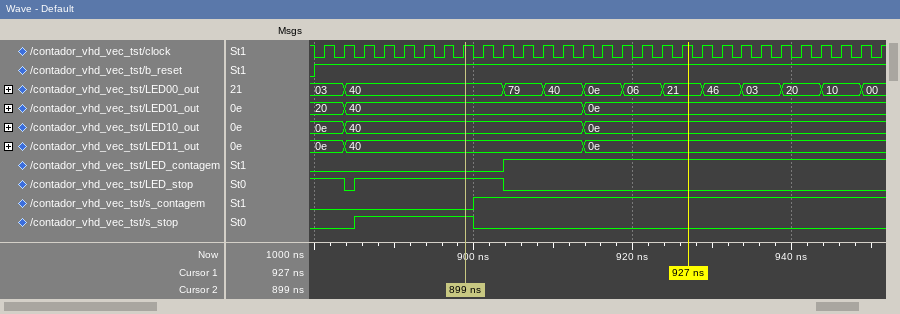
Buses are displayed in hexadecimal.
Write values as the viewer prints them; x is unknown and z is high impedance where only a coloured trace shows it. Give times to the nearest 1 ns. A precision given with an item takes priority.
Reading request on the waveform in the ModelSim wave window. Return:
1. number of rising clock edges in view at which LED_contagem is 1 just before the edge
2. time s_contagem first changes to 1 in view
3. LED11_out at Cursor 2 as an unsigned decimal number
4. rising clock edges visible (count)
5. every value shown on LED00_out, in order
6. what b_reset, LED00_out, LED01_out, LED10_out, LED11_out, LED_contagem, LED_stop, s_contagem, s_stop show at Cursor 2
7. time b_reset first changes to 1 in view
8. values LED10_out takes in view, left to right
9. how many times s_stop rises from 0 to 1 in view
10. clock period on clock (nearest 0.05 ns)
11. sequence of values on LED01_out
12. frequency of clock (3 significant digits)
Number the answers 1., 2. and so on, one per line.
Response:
1. 19
2. 900 ns
3. 64
4. 29
5. 03, 40, 79, 40, 0e, 06, 21, 46, 03, 20, 10, 00
6. b_reset=1, LED00_out=40, LED01_out=40, LED10_out=40, LED11_out=40, LED_contagem=0, LED_stop=1, s_contagem=0, s_stop=1
7. 880 ns
8. 0e, 40, 0e
9. 1
10. 2.5 ns
11. 20, 40, 0e
12. 400 MHz
